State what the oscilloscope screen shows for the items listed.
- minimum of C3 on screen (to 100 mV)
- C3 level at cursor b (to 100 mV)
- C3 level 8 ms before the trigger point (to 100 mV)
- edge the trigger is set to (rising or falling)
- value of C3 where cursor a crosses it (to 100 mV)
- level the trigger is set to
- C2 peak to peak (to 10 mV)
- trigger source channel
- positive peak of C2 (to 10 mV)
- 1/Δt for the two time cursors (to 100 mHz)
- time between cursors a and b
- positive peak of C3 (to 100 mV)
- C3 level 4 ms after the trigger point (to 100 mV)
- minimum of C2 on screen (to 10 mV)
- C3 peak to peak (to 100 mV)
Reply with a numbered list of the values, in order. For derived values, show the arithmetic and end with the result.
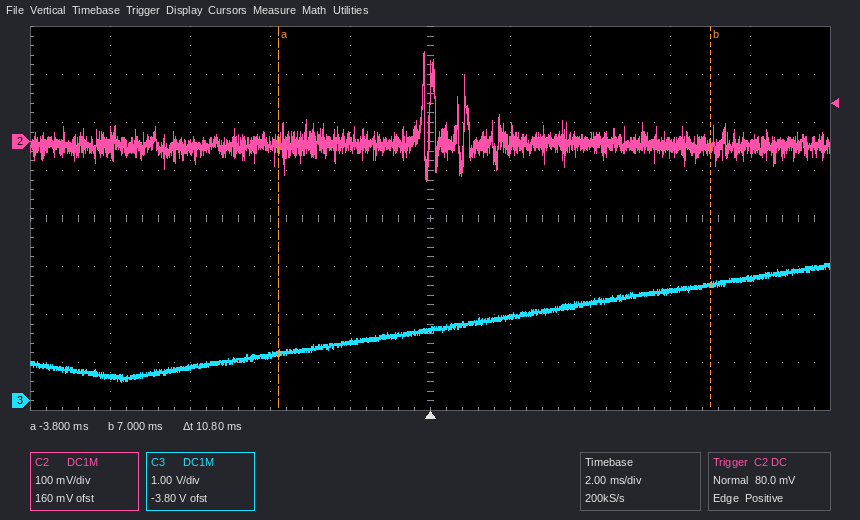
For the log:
1. 400 mV
2. 2.4 V
3. 500 mV
4. rising
5. 1.0 V
6. 80.0 mV
7. 190 mV − (-80 mV) = 270 mV
8. C2
9. 190 mV
10. 1 / 10.8 ms ≈ 92.6 Hz
11. 10.8 ms
12. 2.9 V
13. 2.0 V
14. -80 mV
15. 2.9 V − (400 mV) = 2.5 V
